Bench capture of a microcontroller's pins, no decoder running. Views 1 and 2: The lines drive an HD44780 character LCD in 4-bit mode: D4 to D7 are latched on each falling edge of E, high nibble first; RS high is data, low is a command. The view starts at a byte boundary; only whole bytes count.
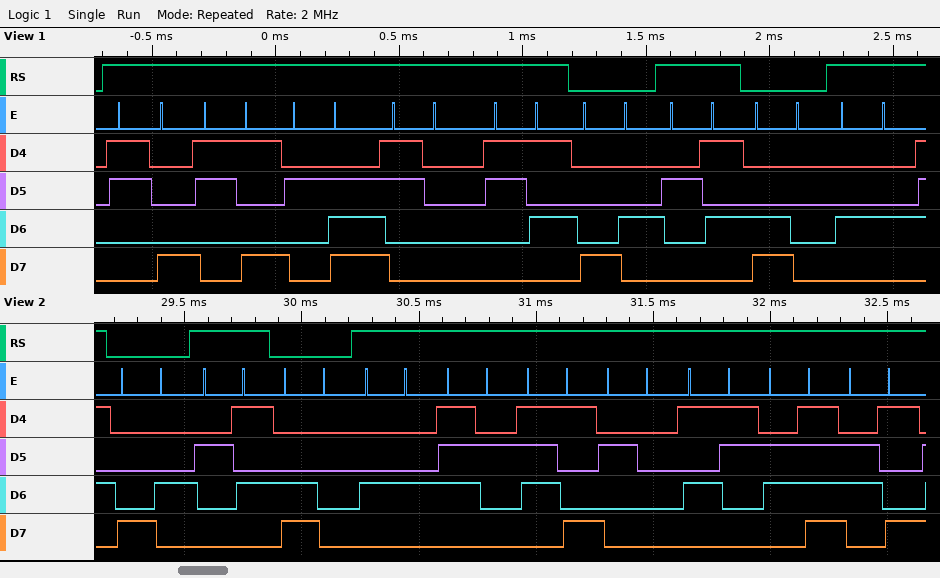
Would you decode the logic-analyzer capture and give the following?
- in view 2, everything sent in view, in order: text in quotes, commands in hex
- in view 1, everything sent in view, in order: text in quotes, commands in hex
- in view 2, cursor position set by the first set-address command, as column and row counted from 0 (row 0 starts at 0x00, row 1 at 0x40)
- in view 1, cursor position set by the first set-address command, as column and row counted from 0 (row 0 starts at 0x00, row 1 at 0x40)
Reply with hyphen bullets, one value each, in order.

- 0x84 "%" 0xC0 "Dry Soi"
- "89.05" 0x84 "%" 0xC0 "D"
- column 4, row 0
- column 4, row 0
